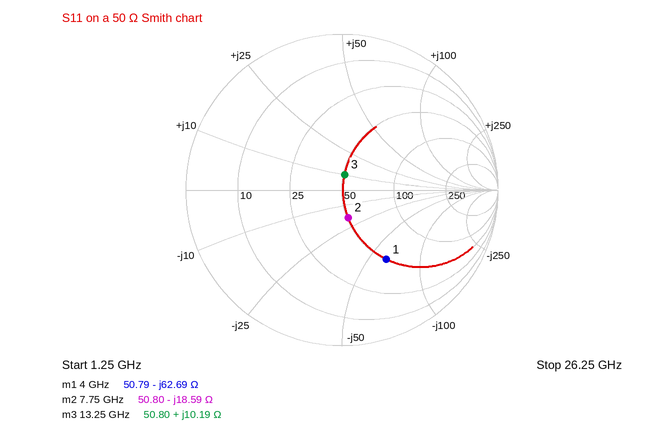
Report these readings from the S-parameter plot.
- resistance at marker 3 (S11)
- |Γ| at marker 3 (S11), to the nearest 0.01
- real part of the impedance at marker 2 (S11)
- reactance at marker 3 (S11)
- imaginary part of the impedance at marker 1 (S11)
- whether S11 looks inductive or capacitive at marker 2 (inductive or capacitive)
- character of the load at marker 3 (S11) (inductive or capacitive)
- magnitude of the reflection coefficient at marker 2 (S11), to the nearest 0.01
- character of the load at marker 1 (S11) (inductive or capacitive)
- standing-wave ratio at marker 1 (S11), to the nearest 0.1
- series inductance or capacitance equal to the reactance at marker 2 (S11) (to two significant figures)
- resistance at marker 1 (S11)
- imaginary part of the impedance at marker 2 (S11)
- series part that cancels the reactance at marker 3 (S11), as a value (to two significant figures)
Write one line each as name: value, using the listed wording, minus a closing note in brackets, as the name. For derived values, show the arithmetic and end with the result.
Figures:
resistance at marker 3: 50.80 Ω
|Γ| at marker 3 (S11), to the nearest 0.01: 0.10
real part of the impedance at marker 2: 50.80 Ω
reactance at marker 3: +10.19 Ω
imaginary part of the impedance at marker 1: -62.69 Ω
whether S11 looks inductive or capacitive at marker 2: capacitive
character of the load at marker 3 (S11): inductive
magnitude of the reflection coefficient at marker 2 (S11), to the nearest 0.01: 0.18
character of the load at marker 1 (S11): capacitive
standing-wave ratio at marker 1 (S11), to the nearest 0.1: 3.2
series inductance or capacitance equal to the reactance at marker 2 (S11): C = 1/(2π × 7.75 GHz × 18.59 Ω) ≈ 1.1 pF
resistance at marker 1: 50.79 Ω
imaginary part of the impedance at marker 2: -18.59 Ω
series part that cancels the reactance at marker 3 (S11), as a value: C = 1/(2π × 13.25 GHz × 10.19 Ω) ≈ 1.2 pF
